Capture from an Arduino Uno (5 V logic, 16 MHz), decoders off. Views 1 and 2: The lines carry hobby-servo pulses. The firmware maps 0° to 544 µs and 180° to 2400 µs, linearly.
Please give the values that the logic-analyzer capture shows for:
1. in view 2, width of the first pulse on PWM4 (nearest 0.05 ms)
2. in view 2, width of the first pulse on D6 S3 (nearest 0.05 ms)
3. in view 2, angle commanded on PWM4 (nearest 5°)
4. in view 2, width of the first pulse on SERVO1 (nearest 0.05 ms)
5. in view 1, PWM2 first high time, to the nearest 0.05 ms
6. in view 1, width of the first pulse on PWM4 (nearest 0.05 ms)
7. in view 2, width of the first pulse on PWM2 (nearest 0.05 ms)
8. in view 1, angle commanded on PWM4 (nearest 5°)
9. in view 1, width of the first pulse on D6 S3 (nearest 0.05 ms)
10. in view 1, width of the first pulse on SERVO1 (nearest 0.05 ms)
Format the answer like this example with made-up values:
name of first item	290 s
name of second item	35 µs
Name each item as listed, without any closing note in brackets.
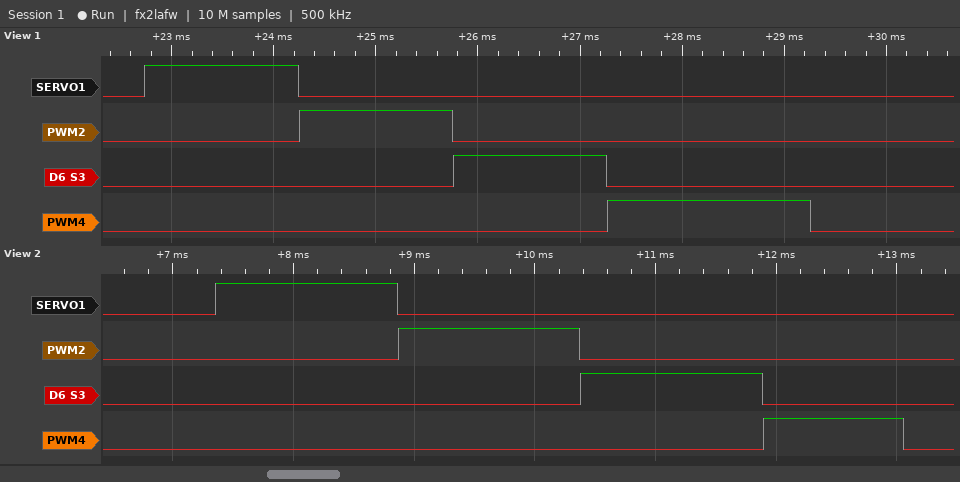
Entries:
in view 2, width of the first pulse on PWM4	1.15 ms
in view 2, width of the first pulse on D6 S3	1.50 ms
in view 2, angle commanded on PWM4	60°
in view 2, width of the first pulse on SERVO1	1.50 ms
in view 1, PWM2 first high time, to the nearest 0.05 ms	1.50 ms
in view 1, width of the first pulse on PWM4	2.00 ms
in view 2, width of the first pulse on PWM2	1.50 ms
in view 1, angle commanded on PWM4	140°
in view 1, width of the first pulse on D6 S3	1.50 ms
in view 1, width of the first pulse on SERVO1	1.50 ms
